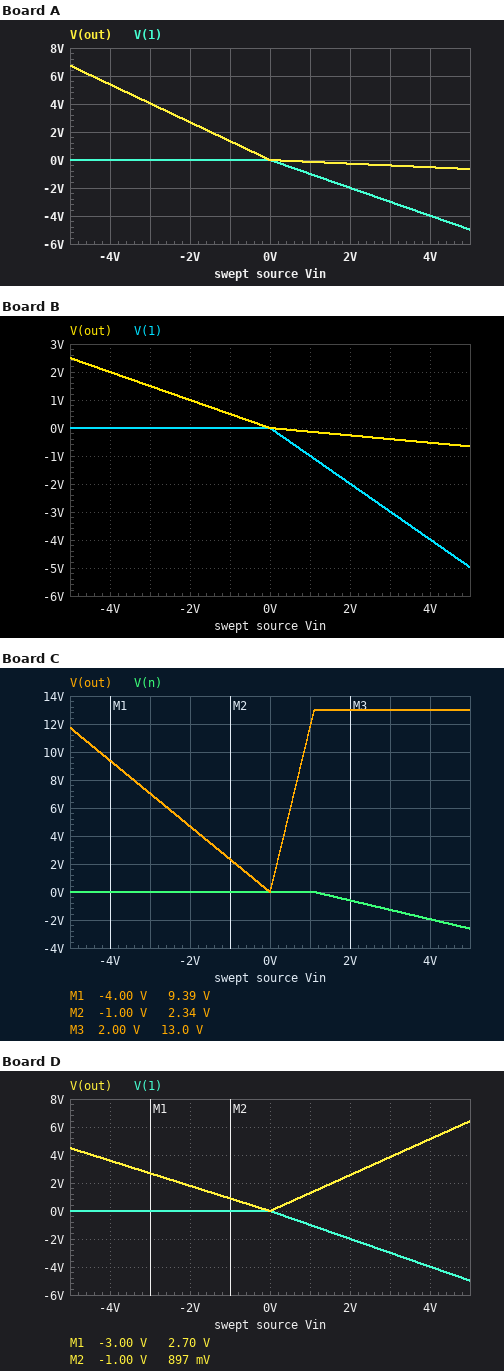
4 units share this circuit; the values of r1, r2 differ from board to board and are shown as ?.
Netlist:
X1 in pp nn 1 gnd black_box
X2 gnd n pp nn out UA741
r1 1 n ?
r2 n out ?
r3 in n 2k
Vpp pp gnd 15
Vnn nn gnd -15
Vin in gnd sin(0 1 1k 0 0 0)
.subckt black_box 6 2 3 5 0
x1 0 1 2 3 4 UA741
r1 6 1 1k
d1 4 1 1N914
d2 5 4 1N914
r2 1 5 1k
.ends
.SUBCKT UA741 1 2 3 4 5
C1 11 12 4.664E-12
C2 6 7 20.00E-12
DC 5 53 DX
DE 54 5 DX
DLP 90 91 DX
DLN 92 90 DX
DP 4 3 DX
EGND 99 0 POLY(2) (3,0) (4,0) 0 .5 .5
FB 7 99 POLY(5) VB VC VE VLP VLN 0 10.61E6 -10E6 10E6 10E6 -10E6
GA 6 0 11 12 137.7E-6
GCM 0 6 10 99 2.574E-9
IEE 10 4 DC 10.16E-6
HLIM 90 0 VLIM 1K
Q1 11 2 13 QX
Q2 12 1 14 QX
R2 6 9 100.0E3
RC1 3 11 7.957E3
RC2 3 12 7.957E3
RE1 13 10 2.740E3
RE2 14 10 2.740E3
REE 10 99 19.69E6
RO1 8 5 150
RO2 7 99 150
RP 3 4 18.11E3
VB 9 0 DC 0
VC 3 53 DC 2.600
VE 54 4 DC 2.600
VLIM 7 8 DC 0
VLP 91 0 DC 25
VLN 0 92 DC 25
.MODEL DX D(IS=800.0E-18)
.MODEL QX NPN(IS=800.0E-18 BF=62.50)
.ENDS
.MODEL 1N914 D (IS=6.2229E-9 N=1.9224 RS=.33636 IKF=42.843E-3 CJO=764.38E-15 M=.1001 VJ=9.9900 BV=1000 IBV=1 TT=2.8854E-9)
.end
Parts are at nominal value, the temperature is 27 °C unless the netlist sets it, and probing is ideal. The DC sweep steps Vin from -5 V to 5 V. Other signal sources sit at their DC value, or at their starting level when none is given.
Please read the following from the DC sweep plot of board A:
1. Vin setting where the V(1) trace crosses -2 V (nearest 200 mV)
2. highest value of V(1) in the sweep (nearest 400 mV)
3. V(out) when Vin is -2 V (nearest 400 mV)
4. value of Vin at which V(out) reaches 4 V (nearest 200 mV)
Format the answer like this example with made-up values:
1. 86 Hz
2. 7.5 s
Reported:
1. 2.0 V
2. 0 V
3. 2.8 V
4. -3.0 V
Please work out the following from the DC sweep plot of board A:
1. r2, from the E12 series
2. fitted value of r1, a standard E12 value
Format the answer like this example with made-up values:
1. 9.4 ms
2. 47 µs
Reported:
1. 2.7 kΩ
2. 2.2 kΩ
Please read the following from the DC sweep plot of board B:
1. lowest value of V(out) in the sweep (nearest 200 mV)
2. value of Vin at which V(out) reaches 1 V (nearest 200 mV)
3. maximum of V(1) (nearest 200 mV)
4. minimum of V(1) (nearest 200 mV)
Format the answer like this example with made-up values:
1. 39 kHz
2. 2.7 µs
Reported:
1. -600 mV
2. -2.0 V
3. 0 V
4. -5.0 V
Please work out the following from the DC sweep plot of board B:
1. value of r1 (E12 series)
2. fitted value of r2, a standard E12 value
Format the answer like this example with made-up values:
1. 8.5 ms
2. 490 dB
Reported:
1. 2.7 kΩ
2. 1 kΩ
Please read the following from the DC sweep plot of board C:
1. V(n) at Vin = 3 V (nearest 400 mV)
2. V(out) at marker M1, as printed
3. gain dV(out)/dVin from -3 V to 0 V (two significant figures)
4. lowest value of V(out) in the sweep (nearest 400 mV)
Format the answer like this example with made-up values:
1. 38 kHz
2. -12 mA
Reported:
1. -1.2 V
2. 9.39 V
3. -2.3 V/V
4. 0 V
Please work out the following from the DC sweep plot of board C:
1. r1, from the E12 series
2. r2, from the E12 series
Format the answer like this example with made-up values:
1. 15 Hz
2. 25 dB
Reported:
1. 330 Ω
2. 4.7 kΩ
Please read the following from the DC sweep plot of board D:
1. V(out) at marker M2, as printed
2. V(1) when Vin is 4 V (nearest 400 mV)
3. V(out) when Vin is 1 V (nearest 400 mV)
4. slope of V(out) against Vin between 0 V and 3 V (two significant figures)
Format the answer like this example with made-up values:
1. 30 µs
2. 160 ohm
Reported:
1. 897 mV
2. -4.0 V
3. 1.2 V
4. 1.3 V/V
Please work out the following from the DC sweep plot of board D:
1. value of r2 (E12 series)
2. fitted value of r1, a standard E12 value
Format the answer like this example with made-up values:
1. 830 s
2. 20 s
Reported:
1. 1.8 kΩ
2. 820 Ω
